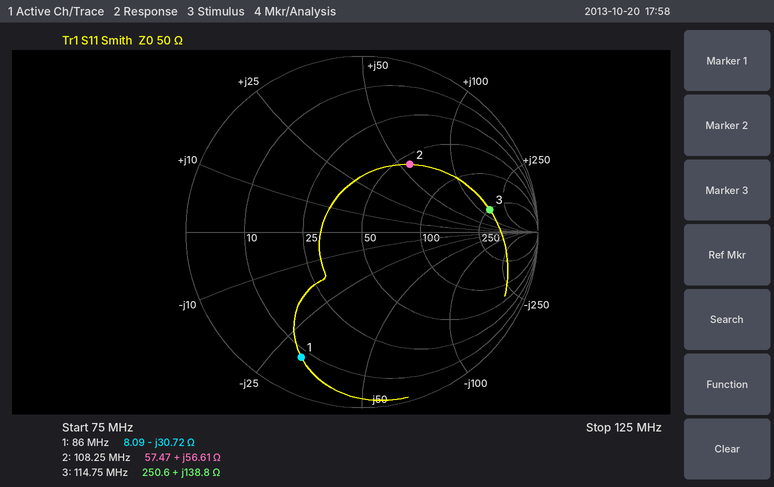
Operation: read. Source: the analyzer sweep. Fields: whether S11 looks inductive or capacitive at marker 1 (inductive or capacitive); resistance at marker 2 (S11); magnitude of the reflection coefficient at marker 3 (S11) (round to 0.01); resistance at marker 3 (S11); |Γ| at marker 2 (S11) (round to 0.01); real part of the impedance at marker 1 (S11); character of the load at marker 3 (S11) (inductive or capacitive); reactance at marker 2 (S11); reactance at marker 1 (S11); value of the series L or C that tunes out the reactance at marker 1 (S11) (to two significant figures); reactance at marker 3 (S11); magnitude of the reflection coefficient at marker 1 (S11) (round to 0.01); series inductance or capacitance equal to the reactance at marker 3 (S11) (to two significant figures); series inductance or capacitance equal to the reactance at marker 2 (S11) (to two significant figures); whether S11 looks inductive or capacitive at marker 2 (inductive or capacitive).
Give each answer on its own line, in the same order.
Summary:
capacitive
57.47 Ω
0.74
250.6 Ω
0.47
8.09 Ω
inductive
+56.61 Ω
-30.72 Ω
57 nH
+138.8 Ω
0.79
190 nH
83 nH
inductive
